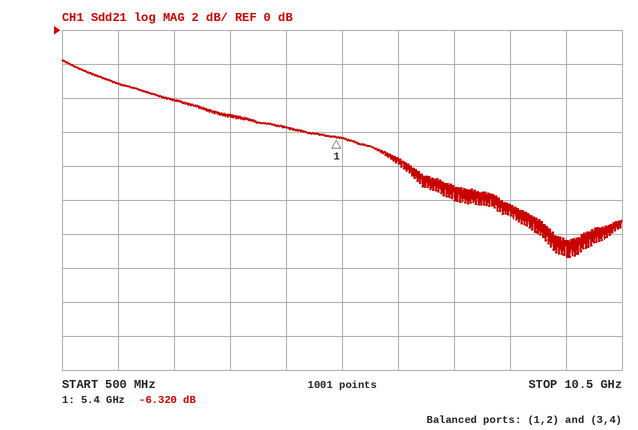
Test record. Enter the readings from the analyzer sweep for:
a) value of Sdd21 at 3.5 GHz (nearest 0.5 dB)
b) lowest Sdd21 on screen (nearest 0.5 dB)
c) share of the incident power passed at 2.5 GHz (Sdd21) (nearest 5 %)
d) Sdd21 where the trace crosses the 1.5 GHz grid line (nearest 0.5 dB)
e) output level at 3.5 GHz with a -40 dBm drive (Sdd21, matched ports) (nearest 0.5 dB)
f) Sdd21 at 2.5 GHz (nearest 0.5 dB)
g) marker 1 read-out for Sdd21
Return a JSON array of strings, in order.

["-5.0 dB", "-13.5 dB", "40 %", "-3.0 dB", "-45.0 dBm", "-4.0 dB", "-6.320 dB"]
